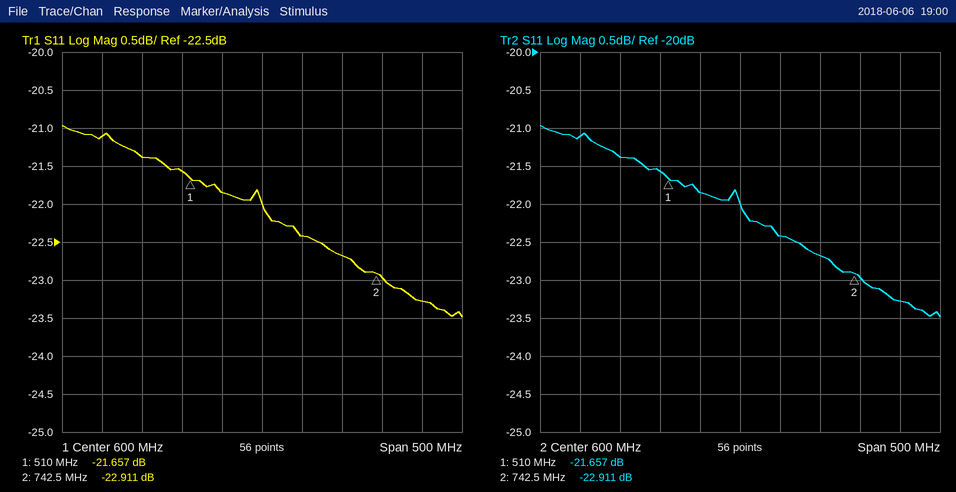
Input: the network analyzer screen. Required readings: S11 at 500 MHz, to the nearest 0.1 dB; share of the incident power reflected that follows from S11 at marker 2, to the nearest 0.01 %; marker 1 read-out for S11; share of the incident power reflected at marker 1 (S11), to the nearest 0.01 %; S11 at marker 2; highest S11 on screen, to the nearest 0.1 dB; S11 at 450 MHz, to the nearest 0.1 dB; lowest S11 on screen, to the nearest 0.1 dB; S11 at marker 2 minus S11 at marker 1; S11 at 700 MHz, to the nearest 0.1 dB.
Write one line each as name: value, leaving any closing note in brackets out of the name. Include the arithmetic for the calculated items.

S11 at 500 MHz, to the nearest 0.1 dB: -21.6 dB
share of the incident power reflected that follows from S11 at marker 2, to the nearest 0.01 %: 10^(-22.911/10) ≈ 0.51 %
marker 1 read-out for S11: -21.657 dB
share of the incident power reflected at marker 1 (S11), to the nearest 0.01 %: 10^(-21.657/10) ≈ 0.68 %
S11 at marker 2: -22.911 dB
highest S11 on screen, to the nearest 0.1 dB: -21.0 dB
S11 at 450 MHz, to the nearest 0.1 dB: -21.4 dB
lowest S11 on screen, to the nearest 0.1 dB: -23.5 dB
S11 at marker 2 minus S11 at marker 1: -22.911 − (-21.657) = -1.254 dB
S11 at 700 MHz, to the nearest 0.1 dB: -22.7 dB
